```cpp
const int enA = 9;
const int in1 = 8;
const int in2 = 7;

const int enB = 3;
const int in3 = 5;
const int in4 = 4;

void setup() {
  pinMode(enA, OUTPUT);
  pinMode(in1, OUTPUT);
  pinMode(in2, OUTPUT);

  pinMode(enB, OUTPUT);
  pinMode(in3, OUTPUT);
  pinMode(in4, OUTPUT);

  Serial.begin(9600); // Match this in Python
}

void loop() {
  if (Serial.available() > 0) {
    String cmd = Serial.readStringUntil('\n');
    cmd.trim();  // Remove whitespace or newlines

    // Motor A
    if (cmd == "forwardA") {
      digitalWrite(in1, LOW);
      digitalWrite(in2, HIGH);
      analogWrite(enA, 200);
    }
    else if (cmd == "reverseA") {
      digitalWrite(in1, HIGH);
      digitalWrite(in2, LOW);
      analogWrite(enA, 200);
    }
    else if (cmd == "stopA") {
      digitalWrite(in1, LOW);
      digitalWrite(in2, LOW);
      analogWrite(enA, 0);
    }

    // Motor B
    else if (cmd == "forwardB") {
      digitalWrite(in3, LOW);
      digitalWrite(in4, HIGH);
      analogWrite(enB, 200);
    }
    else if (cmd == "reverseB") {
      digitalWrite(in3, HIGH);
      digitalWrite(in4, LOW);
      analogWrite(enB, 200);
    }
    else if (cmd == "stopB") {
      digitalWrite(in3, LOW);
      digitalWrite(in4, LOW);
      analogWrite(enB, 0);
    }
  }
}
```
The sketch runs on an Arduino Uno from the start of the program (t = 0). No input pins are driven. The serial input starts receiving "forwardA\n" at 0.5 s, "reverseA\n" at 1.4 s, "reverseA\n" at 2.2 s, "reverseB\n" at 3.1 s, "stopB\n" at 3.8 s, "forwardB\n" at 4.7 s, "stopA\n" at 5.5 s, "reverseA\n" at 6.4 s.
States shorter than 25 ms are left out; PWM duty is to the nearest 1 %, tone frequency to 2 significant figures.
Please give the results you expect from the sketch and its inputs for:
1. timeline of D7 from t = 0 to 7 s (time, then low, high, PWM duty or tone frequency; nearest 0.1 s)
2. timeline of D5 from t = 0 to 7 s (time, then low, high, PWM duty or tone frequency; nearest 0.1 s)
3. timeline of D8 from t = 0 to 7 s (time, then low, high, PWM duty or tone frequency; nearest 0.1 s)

0 s low; 0.5 s high; 1.4 s low
0 s low; 3.1 s high; 3.8 s low
0 s low; 1.4 s high; 5.5 s low; 6.4 s high
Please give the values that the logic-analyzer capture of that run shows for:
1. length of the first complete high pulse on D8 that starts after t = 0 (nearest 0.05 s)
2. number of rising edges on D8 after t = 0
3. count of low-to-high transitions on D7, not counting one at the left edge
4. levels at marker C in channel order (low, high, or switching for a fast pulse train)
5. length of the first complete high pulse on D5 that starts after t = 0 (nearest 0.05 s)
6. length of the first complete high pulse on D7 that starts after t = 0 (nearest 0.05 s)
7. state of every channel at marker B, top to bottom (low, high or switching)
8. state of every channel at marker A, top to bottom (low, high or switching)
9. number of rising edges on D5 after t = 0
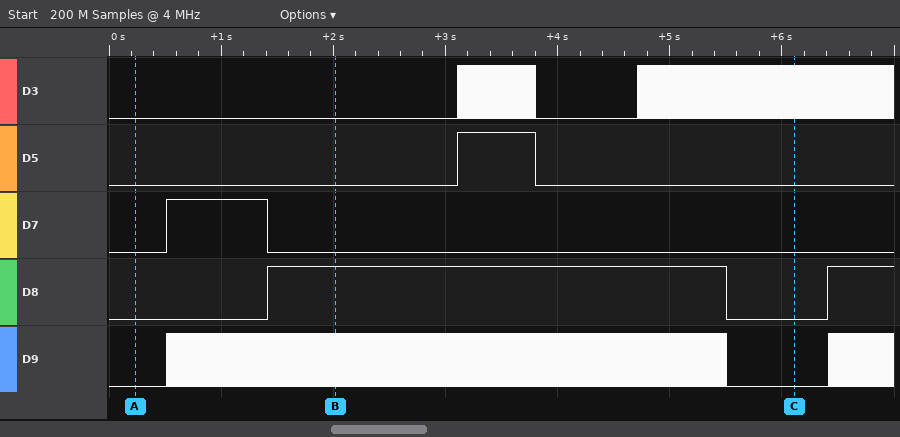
4.10 s
2
1
D3 switching, D5 low, D7 low, D8 low, D9 low
0.70 s
0.90 s
D3 low, D5 low, D7 low, D8 high, D9 switching
D3 low, D5 low, D7 low, D8 low, D9 low
1
